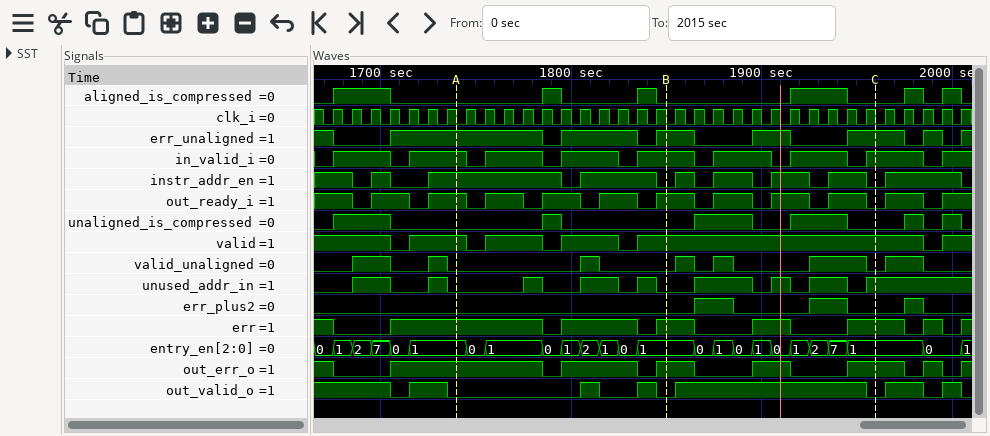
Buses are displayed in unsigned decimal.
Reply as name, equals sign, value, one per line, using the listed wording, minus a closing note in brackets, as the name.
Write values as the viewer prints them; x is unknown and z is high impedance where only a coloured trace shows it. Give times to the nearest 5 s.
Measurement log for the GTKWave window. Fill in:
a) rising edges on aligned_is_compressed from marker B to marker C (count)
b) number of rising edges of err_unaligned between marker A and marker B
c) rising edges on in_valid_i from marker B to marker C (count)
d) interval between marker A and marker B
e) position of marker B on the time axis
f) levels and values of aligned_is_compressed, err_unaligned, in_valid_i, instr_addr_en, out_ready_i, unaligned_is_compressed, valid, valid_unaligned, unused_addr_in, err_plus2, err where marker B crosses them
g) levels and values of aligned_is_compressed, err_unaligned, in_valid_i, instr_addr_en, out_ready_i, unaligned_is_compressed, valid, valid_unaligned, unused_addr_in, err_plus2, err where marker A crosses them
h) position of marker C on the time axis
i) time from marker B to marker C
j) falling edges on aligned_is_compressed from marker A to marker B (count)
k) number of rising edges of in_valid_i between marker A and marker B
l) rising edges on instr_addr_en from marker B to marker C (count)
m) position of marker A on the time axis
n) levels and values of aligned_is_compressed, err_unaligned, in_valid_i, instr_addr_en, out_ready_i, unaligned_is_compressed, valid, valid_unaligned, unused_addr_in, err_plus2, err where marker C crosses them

rising edges on aligned_is_compressed from marker B to marker C = 1
number of rising edges of err_unaligned between marker A and marker B = 2
rising edges on in_valid_i from marker B to marker C = 3
interval between marker A and marker B = 110 s
position of marker B on the time axis = 1850 s
levels and values of aligned_is_compressed, err_unaligned, in_valid_i, instr_addr_en, out_ready_i, unaligned_is_compressed, valid, valid_unaligned, unused_addr_in, err_plus2, err where marker B crosses them = aligned_is_compressed=0, err_unaligned=1, in_valid_i=1, instr_addr_en=0, out_ready_i=1, unaligned_is_compressed=0, valid=1, valid_unaligned=0, unused_addr_in=0, err_plus2=0, err=1
levels and values of aligned_is_compressed, err_unaligned, in_valid_i, instr_addr_en, out_ready_i, unaligned_is_compressed, valid, valid_unaligned, unused_addr_in, err_plus2, err where marker A crosses them = aligned_is_compressed=0, err_unaligned=1, in_valid_i=1, instr_addr_en=1, out_ready_i=1, unaligned_is_compressed=0, valid=1, valid_unaligned=0, unused_addr_in=0, err_plus2=0, err=1
position of marker C on the time axis = 1960 s
time from marker B to marker C = 110 s
falling edges on aligned_is_compressed from marker A to marker B = 2
number of rising edges of in_valid_i between marker A and marker B = 3
rising edges on instr_addr_en from marker B to marker C = 4
position of marker A on the time axis = 1740 s
levels and values of aligned_is_compressed, err_unaligned, in_valid_i, instr_addr_en, out_ready_i, unaligned_is_compressed, valid, valid_unaligned, unused_addr_in, err_plus2, err where marker C crosses them = aligned_is_compressed=0, err_unaligned=1, in_valid_i=1, instr_addr_en=0, out_ready_i=0, unaligned_is_compressed=0, valid=1, valid_unaligned=0, unused_addr_in=1, err_plus2=0, err=1
